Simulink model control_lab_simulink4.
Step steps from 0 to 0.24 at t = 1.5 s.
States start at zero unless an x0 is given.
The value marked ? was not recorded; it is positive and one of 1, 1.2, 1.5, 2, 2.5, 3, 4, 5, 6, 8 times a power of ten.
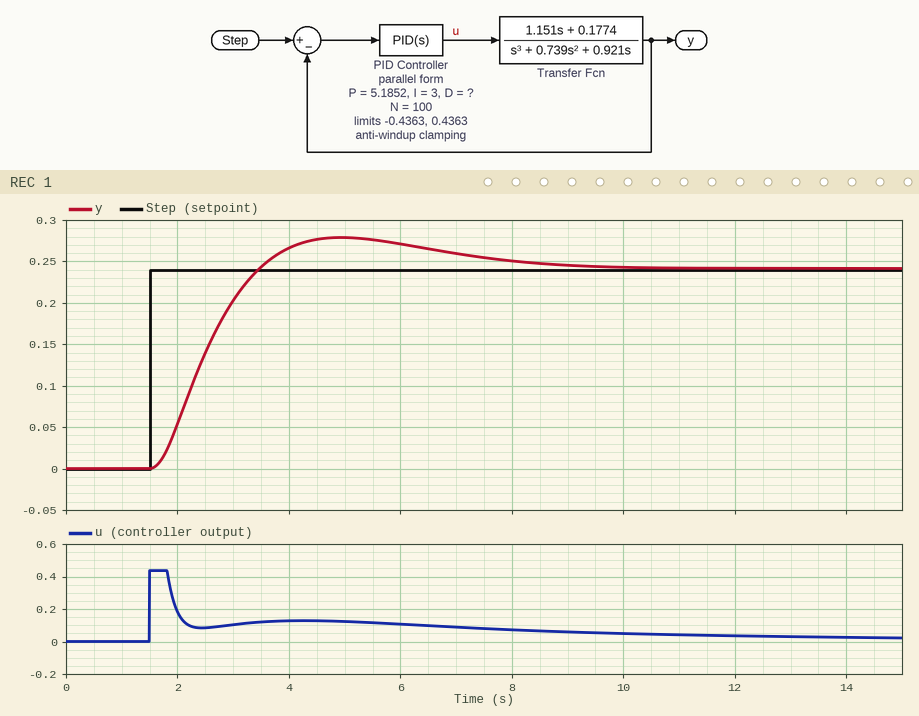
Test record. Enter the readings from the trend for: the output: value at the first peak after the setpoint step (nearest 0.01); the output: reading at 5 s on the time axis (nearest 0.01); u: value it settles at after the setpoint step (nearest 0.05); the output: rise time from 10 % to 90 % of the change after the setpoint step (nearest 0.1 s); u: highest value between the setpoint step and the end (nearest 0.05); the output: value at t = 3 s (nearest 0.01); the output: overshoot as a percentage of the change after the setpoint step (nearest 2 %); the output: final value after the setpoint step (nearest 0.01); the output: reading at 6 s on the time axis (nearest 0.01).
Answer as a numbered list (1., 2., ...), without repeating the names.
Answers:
1. 0.28
2. 0.28
3. 0.00
4. 1.3 s
5. 0.45
6. 0.20
7. 16 %
8. 0.24
9. 0.27
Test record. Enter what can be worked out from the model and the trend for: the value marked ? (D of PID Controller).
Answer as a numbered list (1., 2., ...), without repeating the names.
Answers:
1. 5
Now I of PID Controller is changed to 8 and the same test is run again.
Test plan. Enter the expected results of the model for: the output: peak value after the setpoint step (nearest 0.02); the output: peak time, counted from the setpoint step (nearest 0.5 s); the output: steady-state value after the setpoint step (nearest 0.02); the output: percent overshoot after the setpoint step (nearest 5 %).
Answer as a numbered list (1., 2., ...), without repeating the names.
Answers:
1. 0.32
2. 2.5 s
3. 0.24
4. 35 %
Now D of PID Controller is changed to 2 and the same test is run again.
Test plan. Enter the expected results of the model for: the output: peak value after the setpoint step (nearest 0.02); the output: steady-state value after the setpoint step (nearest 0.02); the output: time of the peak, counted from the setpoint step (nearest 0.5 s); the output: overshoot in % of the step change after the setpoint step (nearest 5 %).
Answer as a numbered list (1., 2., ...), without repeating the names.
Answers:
1. 0.26
2. 0.24
3. 2.0 s
4. 10 %
